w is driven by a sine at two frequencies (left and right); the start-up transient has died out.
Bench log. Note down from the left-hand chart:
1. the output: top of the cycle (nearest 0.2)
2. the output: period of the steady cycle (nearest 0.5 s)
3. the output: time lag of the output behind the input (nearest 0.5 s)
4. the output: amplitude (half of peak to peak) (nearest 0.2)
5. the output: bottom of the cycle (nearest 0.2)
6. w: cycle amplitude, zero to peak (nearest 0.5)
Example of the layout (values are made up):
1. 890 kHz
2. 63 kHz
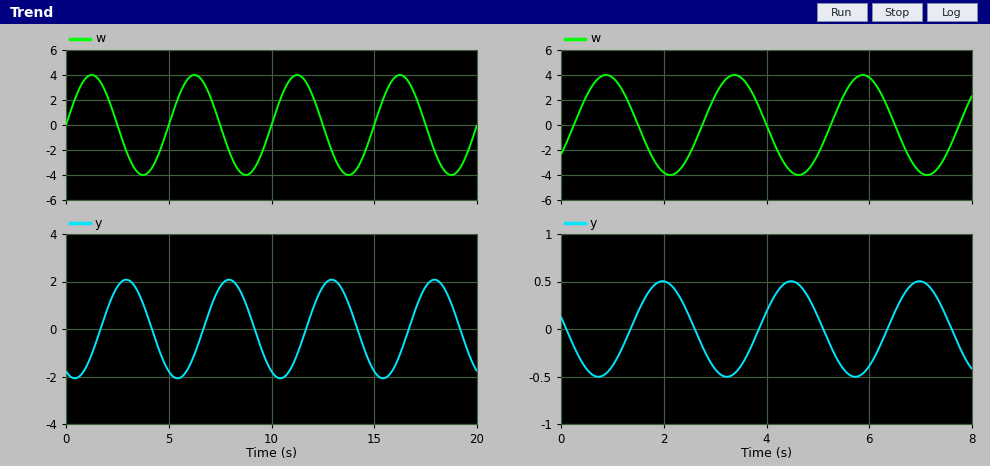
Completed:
1. 2.0
2. 5.0 s
3. 1.5 s
4. 2.0
5. -2.0
6. 4.0
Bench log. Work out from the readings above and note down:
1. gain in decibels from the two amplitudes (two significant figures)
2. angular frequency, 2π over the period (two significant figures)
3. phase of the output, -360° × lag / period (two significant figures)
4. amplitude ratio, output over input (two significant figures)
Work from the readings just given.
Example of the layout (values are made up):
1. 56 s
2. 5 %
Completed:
1. -6.0 dB
2. 1.3 rad/s
3. -110°
4. 0.50
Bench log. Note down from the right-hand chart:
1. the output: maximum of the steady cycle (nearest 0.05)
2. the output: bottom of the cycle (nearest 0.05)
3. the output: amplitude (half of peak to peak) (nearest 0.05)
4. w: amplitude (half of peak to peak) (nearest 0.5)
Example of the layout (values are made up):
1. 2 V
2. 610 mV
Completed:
1. 0.50
2. -0.50
3. 0.50
4. 4.0
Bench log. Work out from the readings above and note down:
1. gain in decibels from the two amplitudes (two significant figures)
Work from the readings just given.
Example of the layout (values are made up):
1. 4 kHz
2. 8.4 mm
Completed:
1. -18 dB
